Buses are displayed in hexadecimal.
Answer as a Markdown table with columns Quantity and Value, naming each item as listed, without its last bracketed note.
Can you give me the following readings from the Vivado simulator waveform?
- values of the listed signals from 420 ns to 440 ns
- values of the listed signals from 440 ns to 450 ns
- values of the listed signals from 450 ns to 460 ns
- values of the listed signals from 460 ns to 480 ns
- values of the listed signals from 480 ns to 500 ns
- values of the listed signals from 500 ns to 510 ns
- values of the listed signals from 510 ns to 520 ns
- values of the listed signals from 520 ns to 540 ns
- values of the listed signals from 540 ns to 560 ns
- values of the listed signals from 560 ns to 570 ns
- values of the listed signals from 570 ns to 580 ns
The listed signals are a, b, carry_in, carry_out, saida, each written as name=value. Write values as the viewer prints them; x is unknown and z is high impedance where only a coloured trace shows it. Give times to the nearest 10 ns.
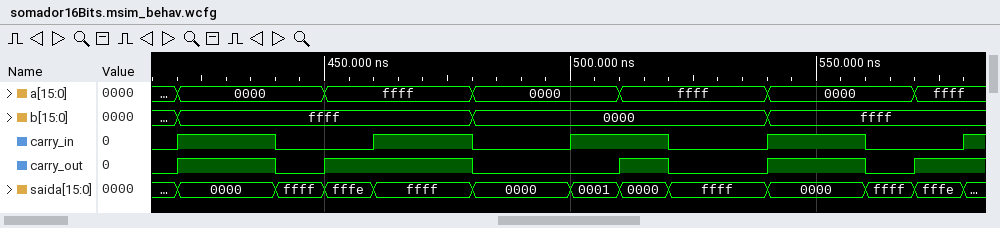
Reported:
| Quantity | Value |
|---|---|
| values of the listed signals from 420 ns to 440 ns | a=0000, b=ffff, carry_in=1, carry_out=1, saida=0000 |
| values of the listed signals from 440 ns to 450 ns | a=0000, b=ffff, carry_in=0, carry_out=0, saida=ffff |
| values of the listed signals from 450 ns to 460 ns | a=ffff, b=ffff, carry_in=0, carry_out=1, saida=fffe |
| values of the listed signals from 460 ns to 480 ns | a=ffff, b=ffff, carry_in=1, carry_out=1, saida=ffff |
| values of the listed signals from 480 ns to 500 ns | a=0000, b=0000, carry_in=0, carry_out=0, saida=0000 |
| values of the listed signals from 500 ns to 510 ns | a=0000, b=0000, carry_in=1, carry_out=0, saida=0001 |
| values of the listed signals from 510 ns to 520 ns | a=ffff, b=0000, carry_in=1, carry_out=1, saida=0000 |
| values of the listed signals from 520 ns to 540 ns | a=ffff, b=0000, carry_in=0, carry_out=0, saida=ffff |
| values of the listed signals from 540 ns to 560 ns | a=0000, b=ffff, carry_in=1, carry_out=1, saida=0000 |
| values of the listed signals from 560 ns to 570 ns | a=0000, b=ffff, carry_in=0, carry_out=0, saida=ffff |
| values of the listed signals from 570 ns to 580 ns | a=ffff, b=ffff, carry_in=0, carry_out=1, saida=fffe |
